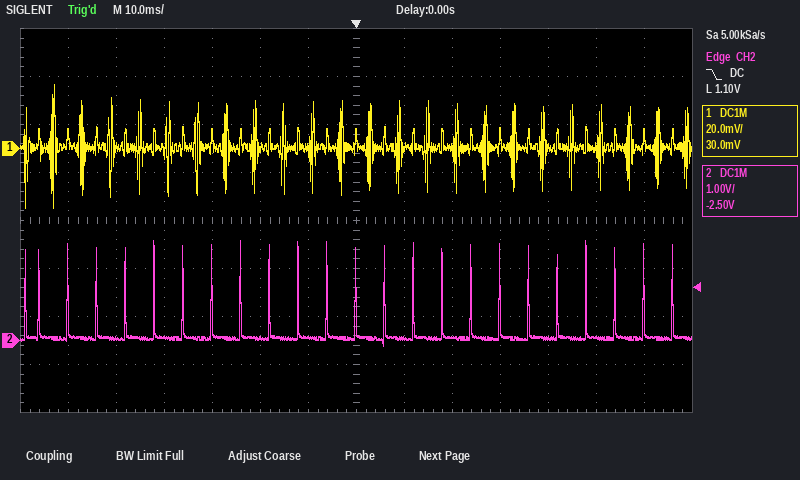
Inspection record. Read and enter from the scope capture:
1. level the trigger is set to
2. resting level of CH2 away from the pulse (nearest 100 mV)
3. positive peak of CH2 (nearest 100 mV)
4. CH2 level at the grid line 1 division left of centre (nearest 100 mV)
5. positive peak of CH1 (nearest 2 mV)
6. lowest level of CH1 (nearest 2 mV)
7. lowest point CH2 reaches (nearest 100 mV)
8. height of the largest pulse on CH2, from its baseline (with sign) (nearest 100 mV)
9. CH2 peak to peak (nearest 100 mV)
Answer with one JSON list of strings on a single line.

["1.10 V", "100 mV", "2.1 V", "100 mV", "26 mV", "-24 mV", "-100 mV", "+2.0 V", "2.2 V"]
